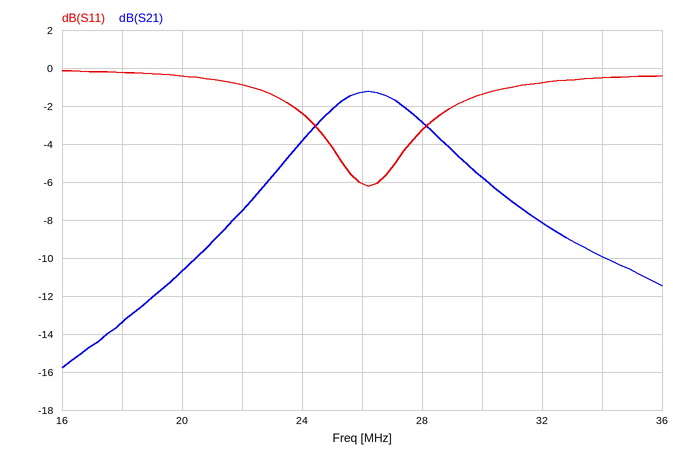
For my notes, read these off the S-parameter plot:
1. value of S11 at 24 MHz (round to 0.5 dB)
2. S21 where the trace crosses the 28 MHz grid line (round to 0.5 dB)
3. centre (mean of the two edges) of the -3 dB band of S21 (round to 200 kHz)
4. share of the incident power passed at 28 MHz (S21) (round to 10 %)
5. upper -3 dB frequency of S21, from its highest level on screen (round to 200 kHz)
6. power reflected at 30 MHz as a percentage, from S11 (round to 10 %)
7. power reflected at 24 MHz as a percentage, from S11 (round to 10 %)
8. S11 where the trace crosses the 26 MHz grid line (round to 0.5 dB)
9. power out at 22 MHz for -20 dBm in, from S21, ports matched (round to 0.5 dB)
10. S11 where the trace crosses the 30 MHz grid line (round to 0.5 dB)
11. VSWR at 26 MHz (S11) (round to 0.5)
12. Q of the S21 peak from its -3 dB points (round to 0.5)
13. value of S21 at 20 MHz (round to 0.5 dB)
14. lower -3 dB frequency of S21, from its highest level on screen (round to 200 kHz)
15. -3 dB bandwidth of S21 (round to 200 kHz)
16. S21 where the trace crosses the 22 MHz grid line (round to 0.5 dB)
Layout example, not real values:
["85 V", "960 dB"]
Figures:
["-2.5 dB", "-3.0 dB", "26.4 MHz", "50 %", "29.0 MHz", "70 %", "60 %", "-6.0 dB", "-27.5 dBm", "-1.5 dB", "3.0", "5.0", "-10.5 dB", "23.8 MHz", "5.2 MHz", "-7.5 dB"]
